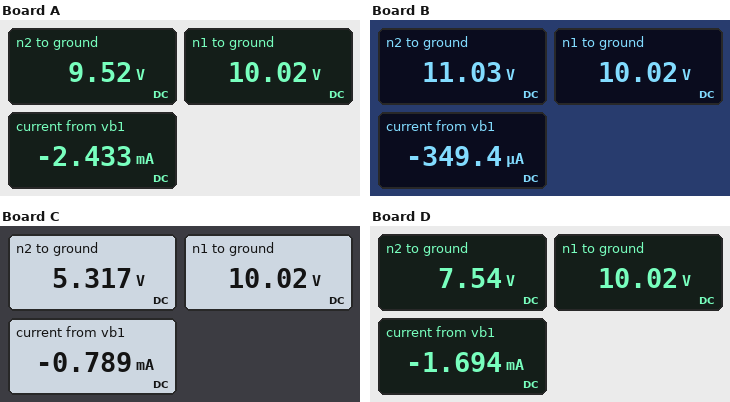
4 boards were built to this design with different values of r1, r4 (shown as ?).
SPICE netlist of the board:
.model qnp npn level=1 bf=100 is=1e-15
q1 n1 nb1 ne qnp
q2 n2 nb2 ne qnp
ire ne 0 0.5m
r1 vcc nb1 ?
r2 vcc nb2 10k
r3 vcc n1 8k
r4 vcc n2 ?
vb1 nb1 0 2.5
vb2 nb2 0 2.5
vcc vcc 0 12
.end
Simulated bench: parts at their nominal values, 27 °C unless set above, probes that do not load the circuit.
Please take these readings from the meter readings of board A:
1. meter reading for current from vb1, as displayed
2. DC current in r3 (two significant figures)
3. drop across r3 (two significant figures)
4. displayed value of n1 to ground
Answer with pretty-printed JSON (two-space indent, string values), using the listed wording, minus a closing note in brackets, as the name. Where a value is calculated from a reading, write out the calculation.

{
  "meter reading for current from vb1, as displayed": "-2.433 mA",
  "DC current in r3": "(12 V - 10.02 V) / 8 kΩ = 250 µA",
  "drop across r3": "12 V - 10.02 V = 2.0 V",
  "displayed value of n1 to ground": "10.02 V"
}
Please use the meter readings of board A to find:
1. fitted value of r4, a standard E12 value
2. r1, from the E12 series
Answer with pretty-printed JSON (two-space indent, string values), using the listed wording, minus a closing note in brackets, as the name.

{
  "fitted value of r4, a standard E12 value": "10 kΩ",
  "r1, from the E12 series": "3.9 kΩ"
}
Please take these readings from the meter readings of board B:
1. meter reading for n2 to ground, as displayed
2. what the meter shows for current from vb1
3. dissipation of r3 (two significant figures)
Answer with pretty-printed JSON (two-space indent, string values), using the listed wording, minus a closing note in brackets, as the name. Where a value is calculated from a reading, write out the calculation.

{
  "meter reading for n2 to ground, as displayed": "11.03 V",
  "what the meter shows for current from vb1": "-349.4 µA",
  "dissipation of r3": "(12 V - 10.02 V)^2 / 8 kΩ = 490 µW"
}
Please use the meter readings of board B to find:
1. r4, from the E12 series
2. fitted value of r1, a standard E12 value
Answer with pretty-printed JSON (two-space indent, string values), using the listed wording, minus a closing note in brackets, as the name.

{
  "r4, from the E12 series": "3.9 kΩ",
  "fitted value of r1, a standard E12 value": "27 kΩ"
}
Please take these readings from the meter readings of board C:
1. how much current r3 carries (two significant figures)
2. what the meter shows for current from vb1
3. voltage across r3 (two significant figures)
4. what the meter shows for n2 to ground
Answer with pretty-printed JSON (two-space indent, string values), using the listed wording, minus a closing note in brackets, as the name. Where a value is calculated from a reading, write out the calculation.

{
  "how much current r3 carries": "(12 V - 10.02 V) / 8 kΩ = 250 µA",
  "what the meter shows for current from vb1": "-0.789 mA",
  "voltage across r3": "12 V - 10.02 V = 2.0 V",
  "what the meter shows for n2 to ground": "5.317 V"
}
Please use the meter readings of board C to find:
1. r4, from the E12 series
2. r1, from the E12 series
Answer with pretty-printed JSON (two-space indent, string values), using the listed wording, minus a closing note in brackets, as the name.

{
  "r4, from the E12 series": "27 kΩ",
  "r1, from the E12 series": "12 kΩ"
}
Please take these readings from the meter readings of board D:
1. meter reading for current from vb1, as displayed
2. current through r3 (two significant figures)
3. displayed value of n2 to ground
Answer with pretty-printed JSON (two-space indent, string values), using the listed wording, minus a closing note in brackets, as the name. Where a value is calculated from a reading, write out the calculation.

{
  "meter reading for current from vb1, as displayed": "-1.694 mA",
  "current through r3": "(12 V - 10.02 V) / 8 kΩ = 250 µA",
  "displayed value of n2 to ground": "7.54 V"
}
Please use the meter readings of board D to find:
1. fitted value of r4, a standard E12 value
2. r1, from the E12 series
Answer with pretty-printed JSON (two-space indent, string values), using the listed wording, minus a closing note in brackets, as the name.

{
  "fitted value of r4, a standard E12 value": "18 kΩ",
  "r1, from the E12 series": "5.6 kΩ"
}
